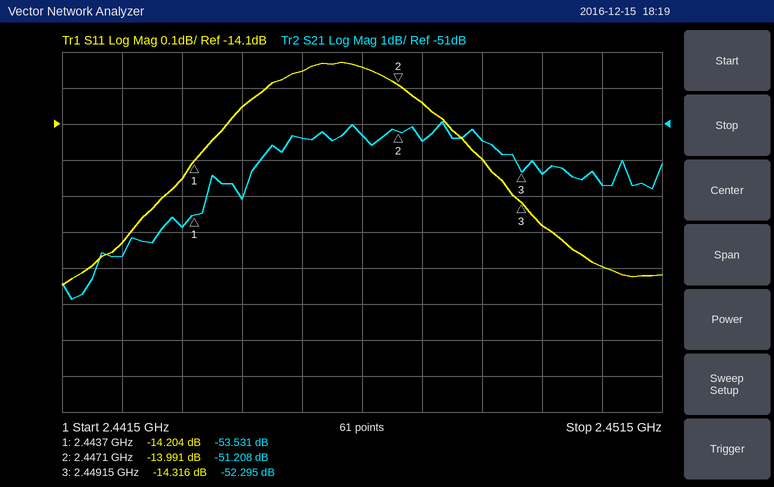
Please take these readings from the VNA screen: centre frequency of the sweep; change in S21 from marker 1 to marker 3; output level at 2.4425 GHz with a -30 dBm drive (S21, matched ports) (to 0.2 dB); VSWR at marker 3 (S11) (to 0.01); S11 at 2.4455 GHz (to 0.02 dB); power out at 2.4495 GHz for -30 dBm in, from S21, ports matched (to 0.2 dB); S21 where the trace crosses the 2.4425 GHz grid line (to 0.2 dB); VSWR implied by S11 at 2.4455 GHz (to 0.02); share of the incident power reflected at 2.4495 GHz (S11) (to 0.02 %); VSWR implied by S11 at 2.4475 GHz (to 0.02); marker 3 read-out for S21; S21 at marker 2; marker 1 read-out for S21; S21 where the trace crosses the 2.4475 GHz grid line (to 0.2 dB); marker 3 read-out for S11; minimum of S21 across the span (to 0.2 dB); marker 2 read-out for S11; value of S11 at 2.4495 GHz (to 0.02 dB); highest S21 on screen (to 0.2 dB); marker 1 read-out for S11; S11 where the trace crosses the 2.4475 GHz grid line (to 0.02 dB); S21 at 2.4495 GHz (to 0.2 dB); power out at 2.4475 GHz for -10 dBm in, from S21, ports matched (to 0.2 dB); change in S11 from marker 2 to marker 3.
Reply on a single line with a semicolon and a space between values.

2.4465 GHz; 1.236 dB; -84.6 dBm; 1.48; -13.96 dB; -82.4 dBm; -54.6 dB; 1.50; 3.64 %; 1.50; -52.295 dB; -51.208 dB; -53.531 dB; -51.4 dB; -14.316 dB; -55.8 dB; -13.991 dB; -14.38 dB; -51.0 dB; -14.204 dB; -14.04 dB; -52.4 dB; -61.4 dBm; -0.325 dB
